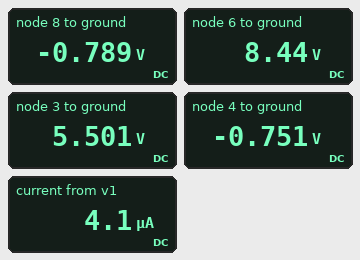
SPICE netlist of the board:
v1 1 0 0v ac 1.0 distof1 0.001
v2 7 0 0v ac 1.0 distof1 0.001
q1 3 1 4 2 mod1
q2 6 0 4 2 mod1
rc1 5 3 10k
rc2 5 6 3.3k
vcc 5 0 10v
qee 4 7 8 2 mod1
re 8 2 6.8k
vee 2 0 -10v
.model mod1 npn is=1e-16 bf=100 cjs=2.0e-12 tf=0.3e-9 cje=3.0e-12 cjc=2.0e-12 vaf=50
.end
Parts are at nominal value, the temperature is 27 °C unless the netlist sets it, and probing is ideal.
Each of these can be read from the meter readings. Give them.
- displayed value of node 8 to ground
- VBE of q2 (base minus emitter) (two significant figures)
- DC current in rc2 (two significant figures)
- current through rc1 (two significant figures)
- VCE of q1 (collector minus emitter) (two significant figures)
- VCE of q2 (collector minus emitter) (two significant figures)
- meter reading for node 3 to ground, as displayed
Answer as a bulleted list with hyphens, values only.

- -0.789 V
- 750 mV
- 470 µA
- 450 µA
- 6.3 V
- 9.2 V
- 5.501 V
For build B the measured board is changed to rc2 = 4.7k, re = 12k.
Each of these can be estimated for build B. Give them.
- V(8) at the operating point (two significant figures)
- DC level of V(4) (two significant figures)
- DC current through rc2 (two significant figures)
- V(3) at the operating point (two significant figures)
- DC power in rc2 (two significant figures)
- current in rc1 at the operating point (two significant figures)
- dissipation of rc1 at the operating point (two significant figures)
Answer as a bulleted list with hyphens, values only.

- -770 mV
- -740 mV
- 270 µA
- 7.4 V
- 330 µW
- 260 µA
- 680 µW
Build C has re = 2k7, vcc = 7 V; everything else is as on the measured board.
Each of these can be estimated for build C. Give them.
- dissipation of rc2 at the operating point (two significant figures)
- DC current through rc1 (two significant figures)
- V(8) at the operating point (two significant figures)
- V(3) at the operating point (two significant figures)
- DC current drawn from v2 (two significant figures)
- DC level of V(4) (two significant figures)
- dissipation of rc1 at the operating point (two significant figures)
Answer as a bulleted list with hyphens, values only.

- 4.9 mW
- 770 µA
- -810 mV
- -730 mV
- 1.2 mA
- -780 mV
- 6.0 mW
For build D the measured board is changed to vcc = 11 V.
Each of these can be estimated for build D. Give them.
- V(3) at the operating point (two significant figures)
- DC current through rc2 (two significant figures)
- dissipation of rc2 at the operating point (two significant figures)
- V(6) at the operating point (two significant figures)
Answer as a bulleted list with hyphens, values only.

- 6.5 V
- 480 µA
- 750 µW
- 9.4 V
